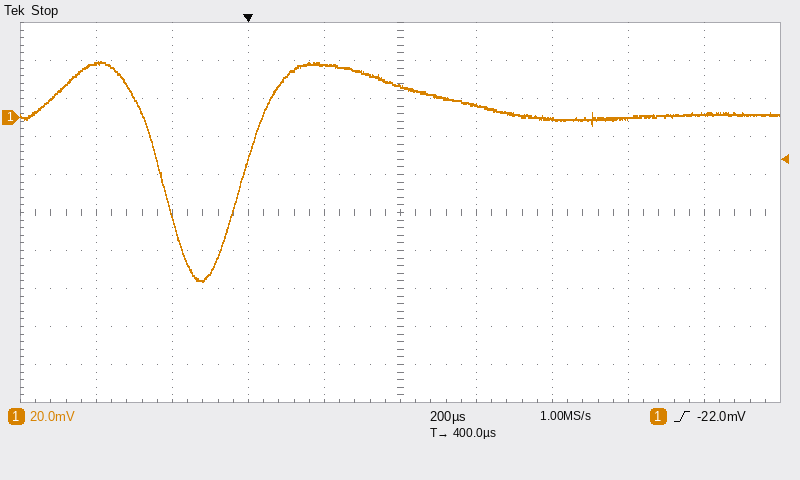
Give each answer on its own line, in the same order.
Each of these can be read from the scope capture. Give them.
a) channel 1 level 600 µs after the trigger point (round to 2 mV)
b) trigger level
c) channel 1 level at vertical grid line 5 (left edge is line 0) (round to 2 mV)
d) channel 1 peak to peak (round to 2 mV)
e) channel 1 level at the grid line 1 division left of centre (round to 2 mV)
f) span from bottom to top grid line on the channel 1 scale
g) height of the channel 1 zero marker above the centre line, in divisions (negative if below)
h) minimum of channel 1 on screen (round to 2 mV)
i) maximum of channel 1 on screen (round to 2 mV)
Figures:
6 mV
-22.0 mV
16 mV
116 mV
28 mV
200 mV
+2.5 div
-86 mV
30 mV
